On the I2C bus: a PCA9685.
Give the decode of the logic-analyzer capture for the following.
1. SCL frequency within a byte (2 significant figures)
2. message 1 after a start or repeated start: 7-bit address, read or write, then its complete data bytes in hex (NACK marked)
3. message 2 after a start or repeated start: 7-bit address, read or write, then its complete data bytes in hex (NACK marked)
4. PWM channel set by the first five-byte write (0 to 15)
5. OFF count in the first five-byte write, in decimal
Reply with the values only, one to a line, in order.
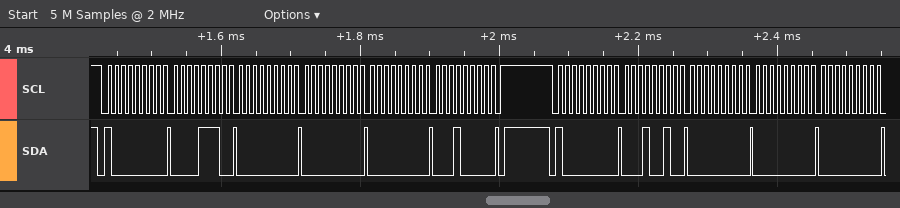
100 kHz
0x40 write: 0E 00 00 00 10
0x40 write: 12 00 00 00
2
4096
